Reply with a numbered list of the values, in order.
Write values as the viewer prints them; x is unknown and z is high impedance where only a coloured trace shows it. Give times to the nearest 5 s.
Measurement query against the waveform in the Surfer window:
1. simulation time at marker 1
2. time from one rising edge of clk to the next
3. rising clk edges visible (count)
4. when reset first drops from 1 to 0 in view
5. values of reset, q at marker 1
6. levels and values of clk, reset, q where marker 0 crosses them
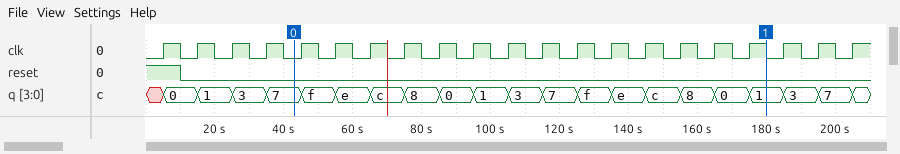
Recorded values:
1. 180 s
2. 10 s
3. 21
4. 10 s
5. reset=0, q=1
6. clk=0, reset=0, q=7
